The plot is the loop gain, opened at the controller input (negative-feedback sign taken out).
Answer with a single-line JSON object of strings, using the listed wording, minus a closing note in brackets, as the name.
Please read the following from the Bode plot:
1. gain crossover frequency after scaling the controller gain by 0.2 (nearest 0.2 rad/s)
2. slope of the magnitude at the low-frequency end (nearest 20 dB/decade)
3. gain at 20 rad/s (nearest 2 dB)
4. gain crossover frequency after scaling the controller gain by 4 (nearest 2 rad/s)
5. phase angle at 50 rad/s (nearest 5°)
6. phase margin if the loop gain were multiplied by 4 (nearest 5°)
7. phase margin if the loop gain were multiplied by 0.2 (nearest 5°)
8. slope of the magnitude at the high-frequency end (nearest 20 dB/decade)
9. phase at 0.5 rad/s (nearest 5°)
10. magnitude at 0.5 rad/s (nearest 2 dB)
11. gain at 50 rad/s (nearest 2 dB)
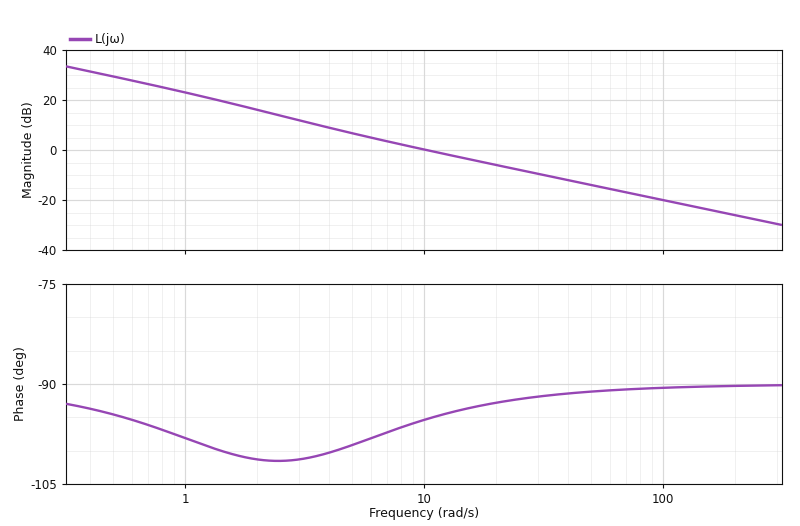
{"gain crossover frequency after scaling the controller gain by 0.2": "2.4 rad/s", "slope of the magnitude at the low-frequency end": "-20 dB/decade", "gain at 20 rad/s": "-6 dB", "gain crossover frequency after scaling the controller gain by 4": "40 rad/s", "phase angle at 50 rad/s": "-90°", "phase margin if the loop gain were multiplied by 4": "90°", "phase margin if the loop gain were multiplied by 0.2": "80°", "slope of the magnitude at the high-frequency end": "-20 dB/decade", "phase at 0.5 rad/s": "-95°", "magnitude at 0.5 rad/s": "30 dB", "gain at 50 rad/s": "-14 dB"}
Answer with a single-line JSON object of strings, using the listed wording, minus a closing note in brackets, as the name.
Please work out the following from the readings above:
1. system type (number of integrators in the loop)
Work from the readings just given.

{"system type": "1"}
